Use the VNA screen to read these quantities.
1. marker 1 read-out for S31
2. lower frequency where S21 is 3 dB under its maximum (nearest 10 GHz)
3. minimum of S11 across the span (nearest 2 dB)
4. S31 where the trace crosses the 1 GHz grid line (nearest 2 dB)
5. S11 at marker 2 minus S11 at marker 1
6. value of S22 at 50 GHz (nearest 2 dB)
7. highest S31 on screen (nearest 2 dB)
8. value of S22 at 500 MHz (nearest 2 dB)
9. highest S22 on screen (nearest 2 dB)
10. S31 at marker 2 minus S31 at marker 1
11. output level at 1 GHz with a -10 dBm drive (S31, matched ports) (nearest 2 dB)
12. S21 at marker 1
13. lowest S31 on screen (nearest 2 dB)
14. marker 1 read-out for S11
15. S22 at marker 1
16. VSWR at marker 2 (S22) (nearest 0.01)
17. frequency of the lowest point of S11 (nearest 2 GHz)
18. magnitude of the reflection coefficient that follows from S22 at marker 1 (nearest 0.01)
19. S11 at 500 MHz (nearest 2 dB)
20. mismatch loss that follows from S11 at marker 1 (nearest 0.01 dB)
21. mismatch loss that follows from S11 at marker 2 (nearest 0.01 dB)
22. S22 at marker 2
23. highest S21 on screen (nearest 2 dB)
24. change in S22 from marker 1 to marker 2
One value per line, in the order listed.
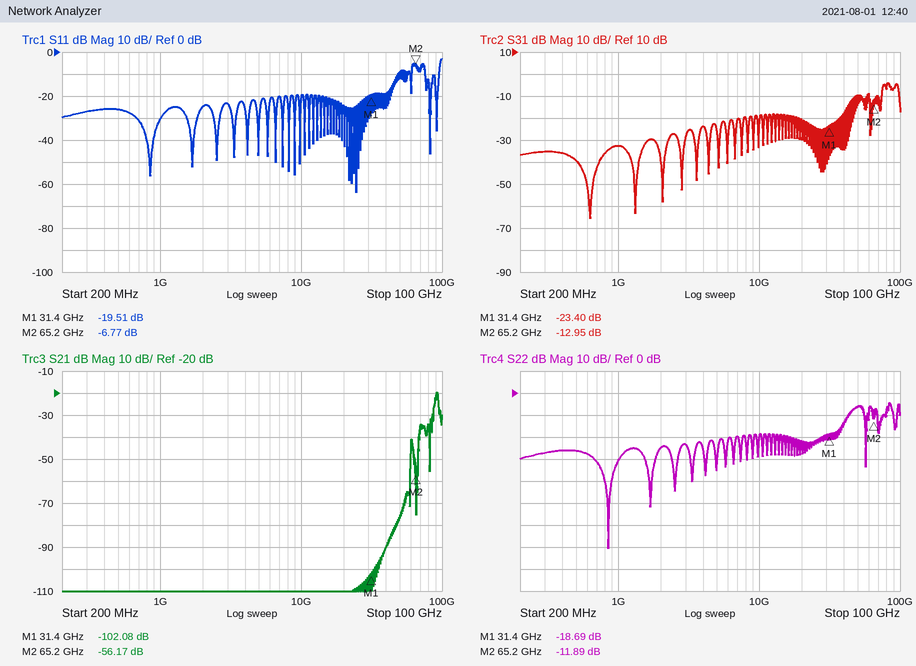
-23.40 dB
90 GHz
-64 dB
-32 dB
12.74 dB
-6 dB
-4 dB
-26 dB
-4 dB
10.45 dB
-42 dBm
-102.08 dB
-66 dB
-19.51 dB
-18.69 dB
1.68
24 GHz
0.12
-26 dB
0.05 dB
1.03 dB
-11.89 dB
-20 dB
6.80 dB
